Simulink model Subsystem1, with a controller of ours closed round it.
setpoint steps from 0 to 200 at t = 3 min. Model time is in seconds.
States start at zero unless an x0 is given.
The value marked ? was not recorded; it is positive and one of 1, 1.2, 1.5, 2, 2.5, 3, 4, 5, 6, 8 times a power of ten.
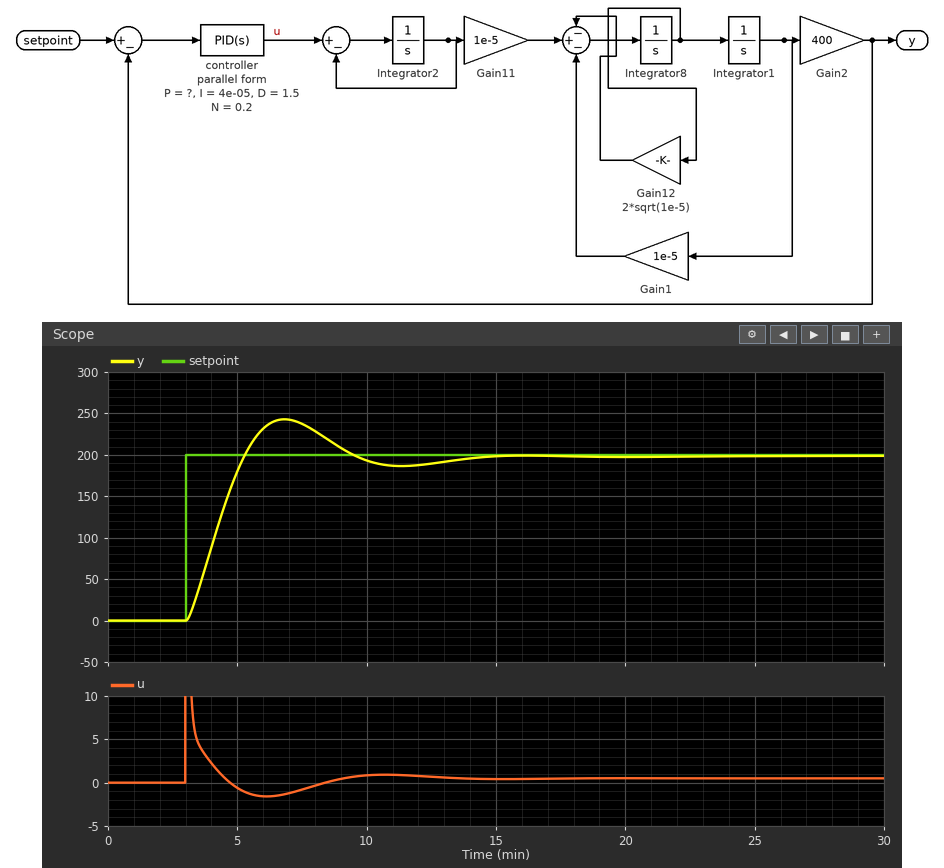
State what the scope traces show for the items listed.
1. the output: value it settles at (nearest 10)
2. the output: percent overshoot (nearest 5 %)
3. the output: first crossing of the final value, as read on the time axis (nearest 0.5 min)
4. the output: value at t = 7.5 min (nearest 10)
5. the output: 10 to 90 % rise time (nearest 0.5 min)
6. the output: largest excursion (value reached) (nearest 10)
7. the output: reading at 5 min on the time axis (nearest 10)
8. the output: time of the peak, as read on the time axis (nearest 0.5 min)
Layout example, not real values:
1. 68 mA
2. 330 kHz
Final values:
1. 200
2. 20 %
3. 5.5 min
4. 240
5. 1.5 min
6. 240
7. 180
8. 7.0 min
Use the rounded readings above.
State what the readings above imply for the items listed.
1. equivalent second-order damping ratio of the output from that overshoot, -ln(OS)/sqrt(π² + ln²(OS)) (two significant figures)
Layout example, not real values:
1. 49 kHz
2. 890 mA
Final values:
1. 0.46
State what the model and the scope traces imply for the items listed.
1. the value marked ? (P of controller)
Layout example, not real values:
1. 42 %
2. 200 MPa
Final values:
1. 0.04
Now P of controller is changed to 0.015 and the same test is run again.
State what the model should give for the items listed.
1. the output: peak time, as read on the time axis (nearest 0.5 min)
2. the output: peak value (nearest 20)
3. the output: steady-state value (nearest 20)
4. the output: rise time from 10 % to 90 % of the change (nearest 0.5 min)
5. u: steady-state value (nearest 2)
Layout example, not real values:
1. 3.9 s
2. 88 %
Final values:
1. 10.5 min
2. 220
3. 200
4. 3.0 min
5. 0
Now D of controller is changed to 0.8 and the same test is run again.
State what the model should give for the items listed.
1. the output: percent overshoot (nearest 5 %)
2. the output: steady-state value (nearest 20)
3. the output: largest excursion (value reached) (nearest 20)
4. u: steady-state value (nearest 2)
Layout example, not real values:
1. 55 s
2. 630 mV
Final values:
1. 30 %
2. 200
3. 260
4. 0
